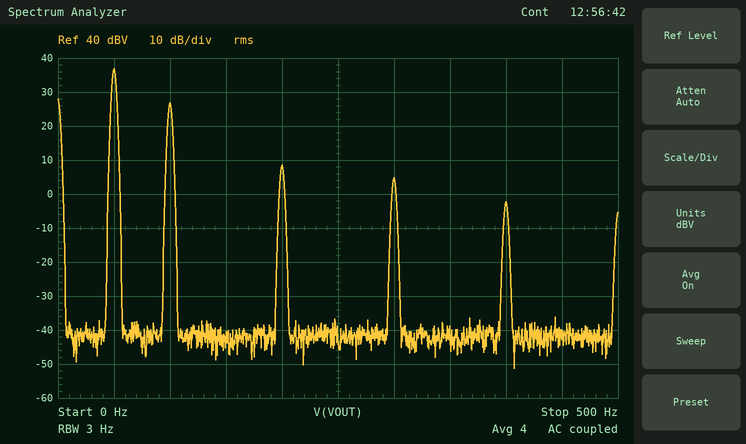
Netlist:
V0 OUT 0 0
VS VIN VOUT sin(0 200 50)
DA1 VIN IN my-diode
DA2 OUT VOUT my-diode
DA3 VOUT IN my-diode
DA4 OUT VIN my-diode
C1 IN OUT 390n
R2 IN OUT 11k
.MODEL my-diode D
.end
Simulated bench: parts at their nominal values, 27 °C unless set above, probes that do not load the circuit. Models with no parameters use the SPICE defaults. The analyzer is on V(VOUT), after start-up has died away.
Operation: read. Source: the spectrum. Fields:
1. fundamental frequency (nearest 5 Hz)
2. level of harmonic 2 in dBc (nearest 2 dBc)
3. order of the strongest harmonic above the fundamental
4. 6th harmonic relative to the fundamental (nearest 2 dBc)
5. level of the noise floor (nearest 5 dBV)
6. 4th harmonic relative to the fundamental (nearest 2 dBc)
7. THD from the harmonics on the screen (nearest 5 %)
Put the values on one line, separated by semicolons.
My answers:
50 Hz; -10 dBc; 2; -32 dBc; -40 dBV; -28 dBc; 30 %
